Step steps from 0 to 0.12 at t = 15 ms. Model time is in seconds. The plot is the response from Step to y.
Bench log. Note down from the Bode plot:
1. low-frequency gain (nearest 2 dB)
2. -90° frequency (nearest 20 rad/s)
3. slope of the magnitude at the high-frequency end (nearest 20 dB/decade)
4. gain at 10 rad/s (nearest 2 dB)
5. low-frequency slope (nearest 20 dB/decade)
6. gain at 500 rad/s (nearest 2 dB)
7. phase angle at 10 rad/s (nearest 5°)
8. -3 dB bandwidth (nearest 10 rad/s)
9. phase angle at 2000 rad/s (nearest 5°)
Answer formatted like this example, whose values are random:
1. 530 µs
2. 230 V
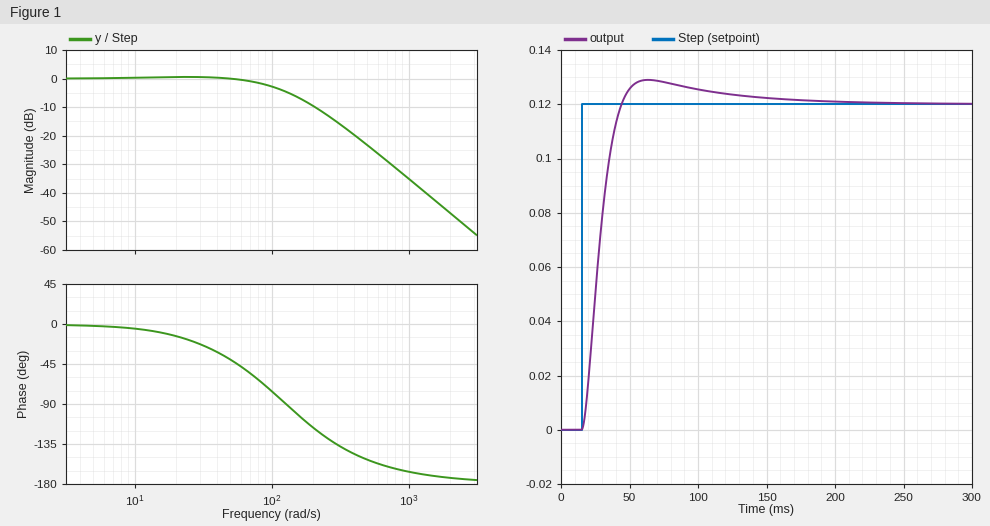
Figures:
1. 0 dB
2. 120 rad/s
3. -40 dB/decade
4. 0 dB
5. 0 dB/decade
6. -24 dB
7. -5°
8. 100 rad/s
9. -175°
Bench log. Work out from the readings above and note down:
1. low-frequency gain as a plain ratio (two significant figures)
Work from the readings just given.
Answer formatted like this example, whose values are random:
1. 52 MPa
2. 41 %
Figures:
1. 1.0
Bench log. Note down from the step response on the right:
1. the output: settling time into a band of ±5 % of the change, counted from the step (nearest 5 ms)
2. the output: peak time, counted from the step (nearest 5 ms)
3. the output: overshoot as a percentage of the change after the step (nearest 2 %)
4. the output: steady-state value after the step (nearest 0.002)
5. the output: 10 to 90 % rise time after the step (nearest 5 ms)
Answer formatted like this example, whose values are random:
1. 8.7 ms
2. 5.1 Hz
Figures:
1. 80 ms
2. 50 ms
3. 8 %
4. 0.120
5. 20 ms
